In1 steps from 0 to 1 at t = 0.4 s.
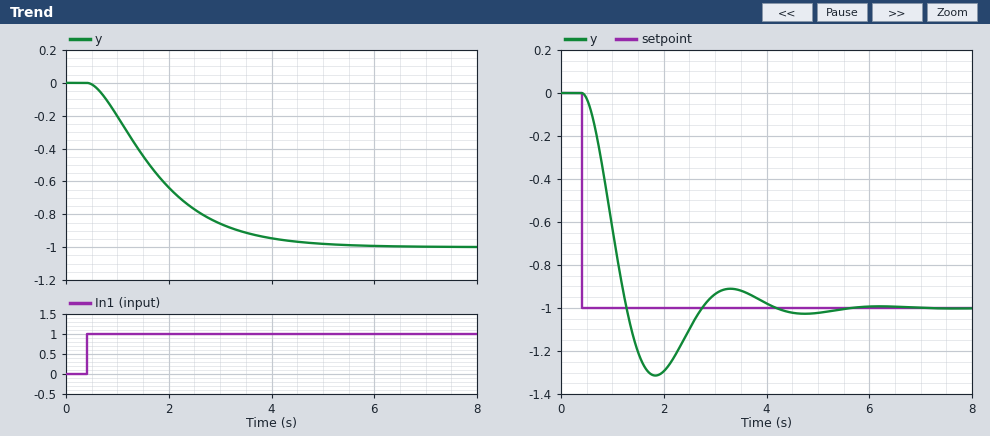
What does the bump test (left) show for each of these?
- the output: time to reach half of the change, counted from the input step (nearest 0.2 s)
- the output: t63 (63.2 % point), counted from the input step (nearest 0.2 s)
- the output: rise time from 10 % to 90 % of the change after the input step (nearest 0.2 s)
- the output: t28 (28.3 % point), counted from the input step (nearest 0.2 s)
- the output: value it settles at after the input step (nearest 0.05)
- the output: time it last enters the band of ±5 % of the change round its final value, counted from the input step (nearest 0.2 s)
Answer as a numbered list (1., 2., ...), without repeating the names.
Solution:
1. 1.2 s
2. 1.6 s
3. 2.6 s
4. 0.8 s
5. -1.00
6. 3.6 s
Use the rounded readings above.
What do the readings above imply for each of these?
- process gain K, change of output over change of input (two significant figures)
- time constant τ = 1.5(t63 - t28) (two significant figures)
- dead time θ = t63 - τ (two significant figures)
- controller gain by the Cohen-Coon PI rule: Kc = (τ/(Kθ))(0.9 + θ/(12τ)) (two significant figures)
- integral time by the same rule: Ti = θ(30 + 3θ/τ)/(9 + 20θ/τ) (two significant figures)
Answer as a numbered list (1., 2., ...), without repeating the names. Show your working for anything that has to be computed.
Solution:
1. (-1 - 0) / 1 = -1.0
2. 1.5 × (1.6 - 0.8) = 1.2 s
3. 1.6 - 1.2 = 0.40 s
4. 1.2 / (-1 × 0.4) × (0.9 + 0.4 / (12 × 1.2)) = -2.8
5. 0.4 × (30 + 3 × 0.4 / 1.2) / (9 + 20 × 0.4 / 1.2) = 0.79 s
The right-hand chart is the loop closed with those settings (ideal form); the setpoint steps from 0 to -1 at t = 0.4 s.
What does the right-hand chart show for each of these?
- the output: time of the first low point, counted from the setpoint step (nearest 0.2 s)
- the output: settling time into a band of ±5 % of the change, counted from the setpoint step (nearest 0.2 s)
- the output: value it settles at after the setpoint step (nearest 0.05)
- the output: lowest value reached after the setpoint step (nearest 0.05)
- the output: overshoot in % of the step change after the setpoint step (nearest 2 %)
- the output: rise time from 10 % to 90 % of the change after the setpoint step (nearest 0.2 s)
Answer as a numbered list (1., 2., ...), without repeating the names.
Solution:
1. 1.4 s
2. 3.4 s
3. -1.00
4. -1.30
5. 32 %
6. 0.6 s
